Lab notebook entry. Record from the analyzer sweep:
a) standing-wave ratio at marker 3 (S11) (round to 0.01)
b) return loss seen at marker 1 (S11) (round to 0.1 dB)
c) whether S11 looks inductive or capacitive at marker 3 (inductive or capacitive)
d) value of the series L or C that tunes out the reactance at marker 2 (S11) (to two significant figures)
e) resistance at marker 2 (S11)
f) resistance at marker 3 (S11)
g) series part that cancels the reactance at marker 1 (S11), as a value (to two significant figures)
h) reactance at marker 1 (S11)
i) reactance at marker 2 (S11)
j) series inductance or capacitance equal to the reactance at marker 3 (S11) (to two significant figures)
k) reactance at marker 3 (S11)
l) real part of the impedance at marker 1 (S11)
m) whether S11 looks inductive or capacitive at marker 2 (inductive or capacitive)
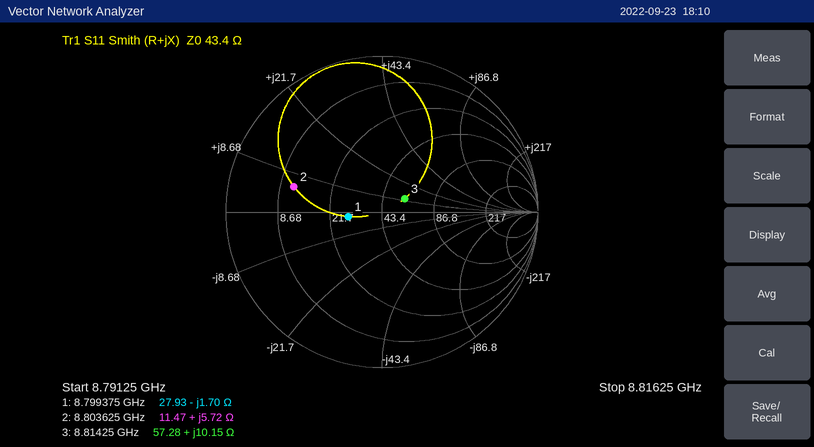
1.41
13.2 dB
inductive
3.2 pF
11.47 Ω
57.28 Ω
31 pH
-1.70 Ω
+5.72 Ω
180 pH
+10.15 Ω
27.93 Ω
inductive
